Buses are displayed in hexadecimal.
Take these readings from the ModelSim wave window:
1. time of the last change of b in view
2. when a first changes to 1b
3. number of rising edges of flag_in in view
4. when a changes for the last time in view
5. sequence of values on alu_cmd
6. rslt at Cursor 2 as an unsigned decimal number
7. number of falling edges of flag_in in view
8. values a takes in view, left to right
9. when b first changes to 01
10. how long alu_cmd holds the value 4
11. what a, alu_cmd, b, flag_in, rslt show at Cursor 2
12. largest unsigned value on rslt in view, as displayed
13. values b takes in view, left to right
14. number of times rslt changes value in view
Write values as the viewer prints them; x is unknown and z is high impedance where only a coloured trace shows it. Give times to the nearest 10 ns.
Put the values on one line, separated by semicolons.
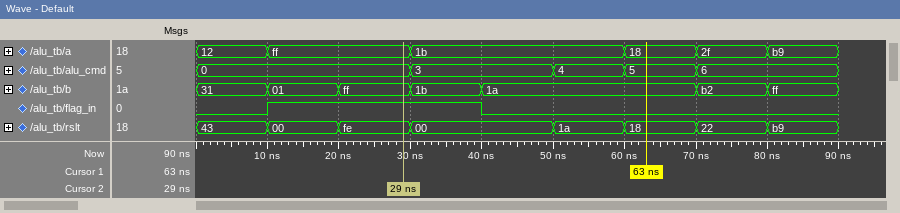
80 ns; 30 ns; 1; 80 ns; 0, 3, 4, 5, 6; 254; 1; 12, ff, 1b, 18, 2f, b9; 10 ns; 10 ns; a=ff, alu_cmd=0, b=ff, flag_in=1, rslt=fe; fe; 31, 01, ff, 1b, 1a, b2, ff; 7
